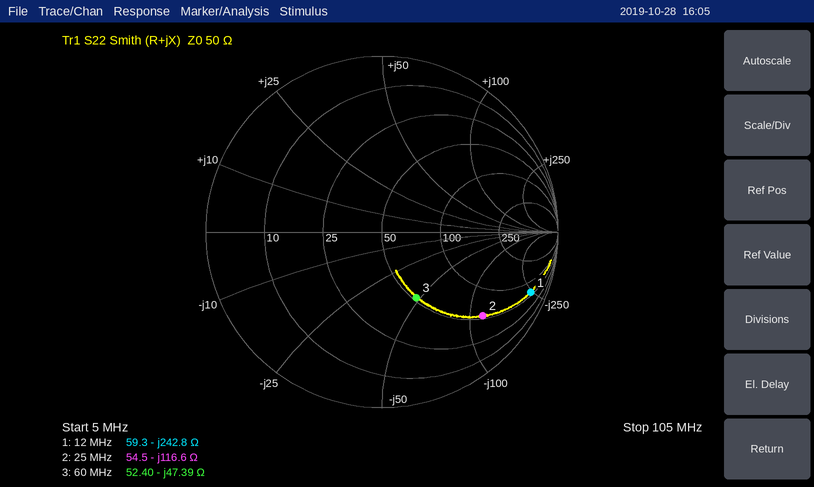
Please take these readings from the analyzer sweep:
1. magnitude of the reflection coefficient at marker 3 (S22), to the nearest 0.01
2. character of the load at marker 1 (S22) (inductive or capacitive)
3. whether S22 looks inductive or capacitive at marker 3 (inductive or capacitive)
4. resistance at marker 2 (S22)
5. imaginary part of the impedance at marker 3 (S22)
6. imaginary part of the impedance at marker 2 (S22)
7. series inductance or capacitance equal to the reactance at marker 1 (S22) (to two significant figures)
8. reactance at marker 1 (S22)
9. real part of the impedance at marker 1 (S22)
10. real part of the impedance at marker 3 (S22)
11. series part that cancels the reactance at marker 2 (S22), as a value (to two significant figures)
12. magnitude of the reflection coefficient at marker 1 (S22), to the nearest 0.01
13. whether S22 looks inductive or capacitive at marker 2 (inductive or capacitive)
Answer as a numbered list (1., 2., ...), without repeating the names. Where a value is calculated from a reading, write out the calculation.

1. 0.42
2. capacitive
3. capacitive
4. 54.5 Ω
5. -47.39 Ω
6. -116.6 Ω
7. C = 1/(2π × 12 MHz × 242.8 Ω) ≈ 55 pF
8. -242.8 Ω
9. 59.3 Ω
10. 52.40 Ω
11. L = 116.6 Ω/(2π × 25 MHz) ≈ 742 nH, so 740 nH to two significant figures
12. 0.91
13. capacitive
